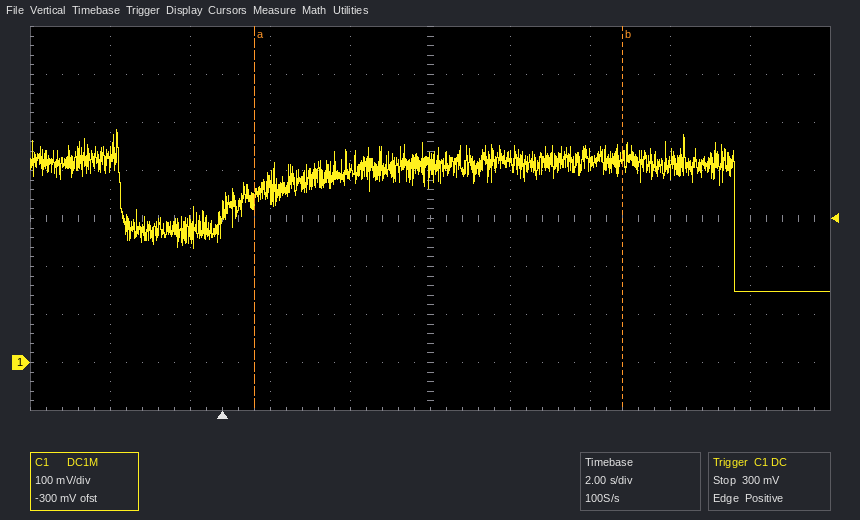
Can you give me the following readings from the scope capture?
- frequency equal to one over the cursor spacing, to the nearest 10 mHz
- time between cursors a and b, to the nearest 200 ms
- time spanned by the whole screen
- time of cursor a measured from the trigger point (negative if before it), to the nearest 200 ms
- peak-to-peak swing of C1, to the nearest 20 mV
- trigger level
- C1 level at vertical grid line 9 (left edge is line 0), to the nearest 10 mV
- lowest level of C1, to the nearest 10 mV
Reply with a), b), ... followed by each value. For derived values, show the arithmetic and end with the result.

a) 1 / 9.2 s ≈ 110 mHz
b) 9.2 s
c) 20 s
d) +800 ms
e) 340 mV
f) 300 mV
g) 150 mV
h) 150 mV
